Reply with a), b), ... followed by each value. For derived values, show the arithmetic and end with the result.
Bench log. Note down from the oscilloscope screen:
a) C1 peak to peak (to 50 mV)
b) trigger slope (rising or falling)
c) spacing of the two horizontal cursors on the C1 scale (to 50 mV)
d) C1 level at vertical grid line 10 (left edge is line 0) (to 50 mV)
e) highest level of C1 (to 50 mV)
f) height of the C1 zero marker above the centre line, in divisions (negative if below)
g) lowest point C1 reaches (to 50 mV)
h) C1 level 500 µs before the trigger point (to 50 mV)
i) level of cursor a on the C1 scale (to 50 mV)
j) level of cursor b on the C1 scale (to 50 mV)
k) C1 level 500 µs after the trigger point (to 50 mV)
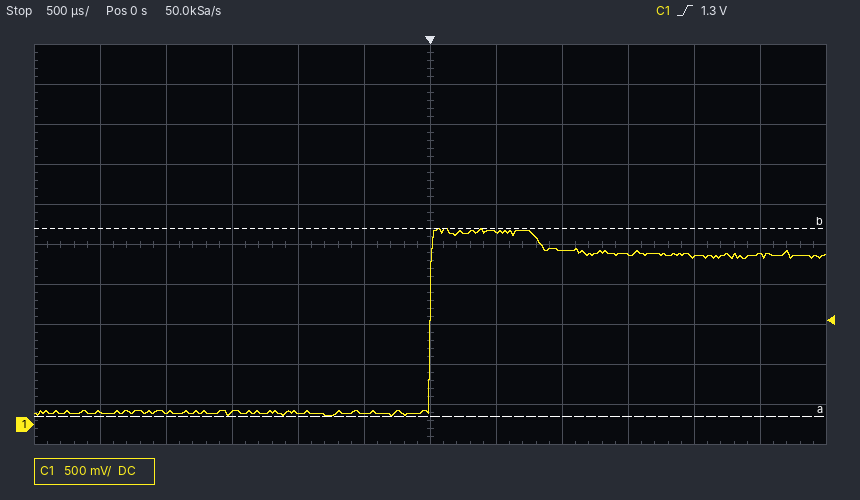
a) 2.45 V − (100 mV) = 2.35 V
b) rising
c) 2.35 V
d) 2.10 V
e) 2.45 V
f) -4.5 div
g) 100 mV
h) 150 mV
i) 100 mV
j) 2.45 V
k) 2.40 V
